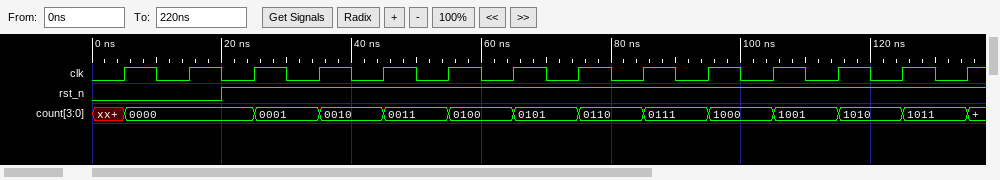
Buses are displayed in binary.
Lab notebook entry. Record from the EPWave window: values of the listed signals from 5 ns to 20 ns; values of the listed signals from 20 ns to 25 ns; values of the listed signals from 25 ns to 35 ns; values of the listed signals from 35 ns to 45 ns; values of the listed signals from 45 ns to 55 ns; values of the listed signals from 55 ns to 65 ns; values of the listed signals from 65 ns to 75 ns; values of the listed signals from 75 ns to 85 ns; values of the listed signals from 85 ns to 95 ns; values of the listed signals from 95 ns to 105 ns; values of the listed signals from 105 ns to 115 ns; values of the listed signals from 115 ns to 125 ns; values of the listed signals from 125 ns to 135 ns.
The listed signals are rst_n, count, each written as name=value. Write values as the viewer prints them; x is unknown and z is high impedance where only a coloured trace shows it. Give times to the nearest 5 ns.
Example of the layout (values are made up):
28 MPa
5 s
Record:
rst_n=0, count=0000
rst_n=1, count=0000
rst_n=1, count=0001
rst_n=1, count=0010
rst_n=1, count=0011
rst_n=1, count=0100
rst_n=1, count=0101
rst_n=1, count=0110
rst_n=1, count=0111
rst_n=1, count=1000
rst_n=1, count=1001
rst_n=1, count=1010
rst_n=1, count=1011
